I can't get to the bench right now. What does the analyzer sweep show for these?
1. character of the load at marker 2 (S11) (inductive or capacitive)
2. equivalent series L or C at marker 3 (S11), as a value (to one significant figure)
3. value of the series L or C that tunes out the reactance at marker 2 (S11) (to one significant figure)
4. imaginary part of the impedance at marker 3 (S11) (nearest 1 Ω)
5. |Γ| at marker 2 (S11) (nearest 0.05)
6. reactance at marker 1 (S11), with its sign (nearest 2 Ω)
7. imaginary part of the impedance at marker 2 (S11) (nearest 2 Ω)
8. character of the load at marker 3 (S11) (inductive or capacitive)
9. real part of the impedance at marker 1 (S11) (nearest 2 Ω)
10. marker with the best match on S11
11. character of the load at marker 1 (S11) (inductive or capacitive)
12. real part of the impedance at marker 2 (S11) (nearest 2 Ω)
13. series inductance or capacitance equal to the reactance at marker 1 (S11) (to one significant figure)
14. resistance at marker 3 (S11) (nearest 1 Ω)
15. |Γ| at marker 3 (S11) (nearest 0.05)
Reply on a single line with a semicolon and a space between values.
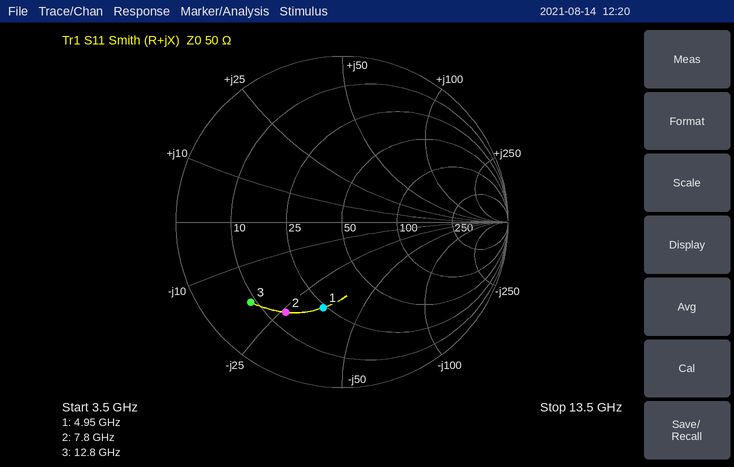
capacitive; 700 fF; 500 pH; -18 Ω; 0.65; -34 Ω; -26 Ω; capacitive; 24 Ω; marker 1; capacitive; 14 Ω; 900 fF; 9 Ω; 0.75
